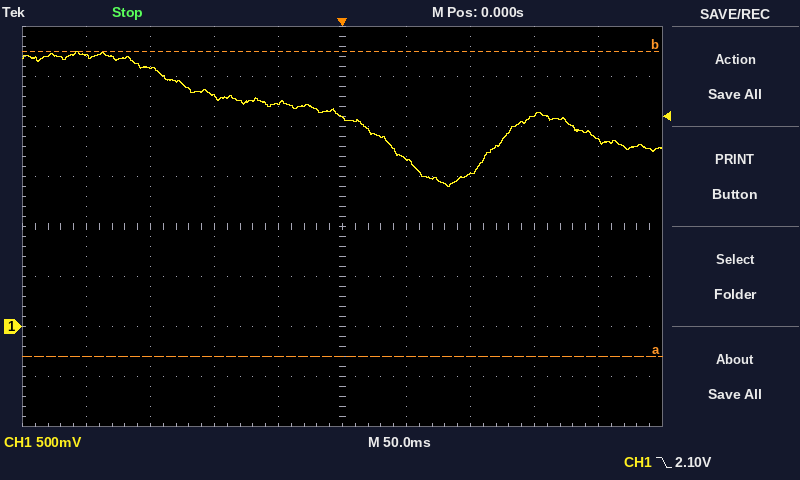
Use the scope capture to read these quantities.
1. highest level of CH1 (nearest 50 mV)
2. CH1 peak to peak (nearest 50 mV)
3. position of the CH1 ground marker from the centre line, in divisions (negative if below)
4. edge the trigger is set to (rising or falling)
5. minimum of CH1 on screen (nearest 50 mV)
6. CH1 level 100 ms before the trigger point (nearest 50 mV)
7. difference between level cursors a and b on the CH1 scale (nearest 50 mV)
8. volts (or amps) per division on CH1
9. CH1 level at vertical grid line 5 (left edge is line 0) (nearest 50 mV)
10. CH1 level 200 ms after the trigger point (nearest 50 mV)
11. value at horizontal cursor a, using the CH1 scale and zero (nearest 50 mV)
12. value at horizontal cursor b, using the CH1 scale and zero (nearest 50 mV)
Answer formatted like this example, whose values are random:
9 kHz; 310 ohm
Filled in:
2.75 V; 1.35 V; -2.0 div; falling; 1.40 V; 2.30 V; 3.05 V; 500 mV; 2.10 V; 1.85 V; -300 mV; 2.75 V
